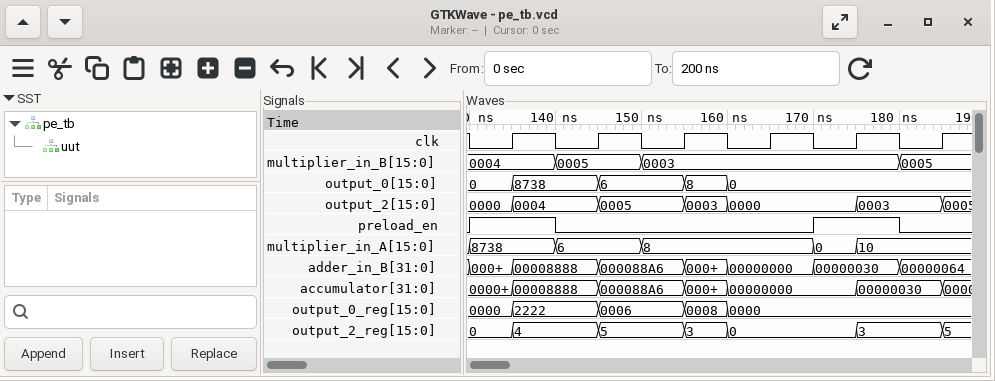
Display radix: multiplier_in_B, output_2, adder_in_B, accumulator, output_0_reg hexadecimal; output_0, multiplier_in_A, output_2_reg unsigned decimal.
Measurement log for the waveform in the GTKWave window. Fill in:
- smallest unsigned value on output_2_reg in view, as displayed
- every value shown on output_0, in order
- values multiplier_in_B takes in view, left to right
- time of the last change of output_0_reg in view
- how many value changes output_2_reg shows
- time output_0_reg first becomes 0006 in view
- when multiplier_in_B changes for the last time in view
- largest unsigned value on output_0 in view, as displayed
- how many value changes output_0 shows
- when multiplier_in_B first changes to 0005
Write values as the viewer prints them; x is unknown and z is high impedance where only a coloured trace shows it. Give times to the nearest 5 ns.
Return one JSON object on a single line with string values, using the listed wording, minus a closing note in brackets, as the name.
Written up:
{"smallest unsigned value on output_2_reg in view, as displayed": "0", "every value shown on output_0, in order": "0, 8738, 6, 8, 0", "values multiplier_in_B takes in view, left to right": "0004, 0005, 0003, 0005", "time of the last change of output_0_reg in view": "160 ns", "how many value changes output_2_reg shows": "6", "time output_0_reg first becomes 0006 in view": "145 ns", "when multiplier_in_B changes for the last time in view": "180 ns", "largest unsigned value on output_0 in view, as displayed": "8738", "how many value changes output_0 shows": "4", "when multiplier_in_B first changes to 0005": "140 ns"}
